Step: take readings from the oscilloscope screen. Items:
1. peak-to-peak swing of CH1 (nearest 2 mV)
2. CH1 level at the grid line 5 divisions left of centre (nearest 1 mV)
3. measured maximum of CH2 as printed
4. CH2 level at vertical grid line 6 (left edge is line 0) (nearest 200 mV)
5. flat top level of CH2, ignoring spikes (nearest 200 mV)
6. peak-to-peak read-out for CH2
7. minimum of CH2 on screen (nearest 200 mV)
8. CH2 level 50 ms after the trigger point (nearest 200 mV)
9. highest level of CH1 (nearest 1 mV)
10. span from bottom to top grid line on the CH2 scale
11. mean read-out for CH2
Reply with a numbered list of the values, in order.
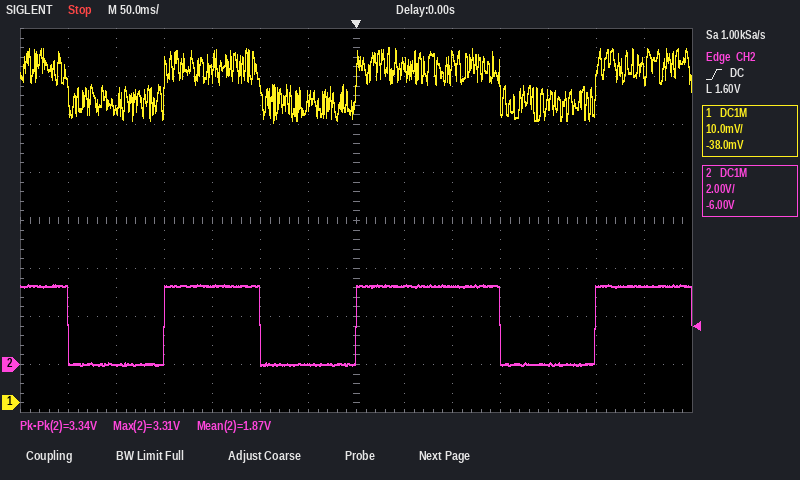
1. 16 mV
2. 61 mV
3. 3.31 V
4. 0.0 V
5. 3.2 V
6. 3.34 V
7. 0.0 V
8. 3.2 V
9. 74 mV
10. 16 V
11. 1.87 V
